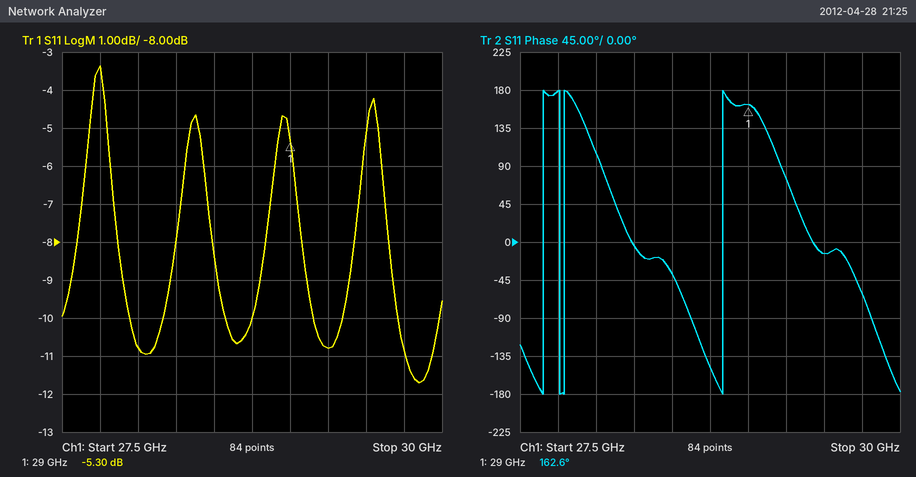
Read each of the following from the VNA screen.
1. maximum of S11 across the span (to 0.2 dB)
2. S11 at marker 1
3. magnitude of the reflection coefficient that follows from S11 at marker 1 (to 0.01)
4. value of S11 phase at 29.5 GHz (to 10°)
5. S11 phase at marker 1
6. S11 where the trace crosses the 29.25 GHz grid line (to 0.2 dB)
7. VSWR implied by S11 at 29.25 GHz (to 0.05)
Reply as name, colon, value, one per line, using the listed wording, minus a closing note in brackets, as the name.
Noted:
maximum of S11 across the span: -3.4 dB
S11 at marker 1: -5.30 dB
magnitude of the reflection coefficient that follows from S11 at marker 1: 0.54
value of S11 phase at 29.5 GHz: -10°
S11 phase at marker 1: 162.6°
S11 where the trace crosses the 29.25 GHz grid line: -10.8 dB
VSWR implied by S11 at 29.25 GHz: 1.80
